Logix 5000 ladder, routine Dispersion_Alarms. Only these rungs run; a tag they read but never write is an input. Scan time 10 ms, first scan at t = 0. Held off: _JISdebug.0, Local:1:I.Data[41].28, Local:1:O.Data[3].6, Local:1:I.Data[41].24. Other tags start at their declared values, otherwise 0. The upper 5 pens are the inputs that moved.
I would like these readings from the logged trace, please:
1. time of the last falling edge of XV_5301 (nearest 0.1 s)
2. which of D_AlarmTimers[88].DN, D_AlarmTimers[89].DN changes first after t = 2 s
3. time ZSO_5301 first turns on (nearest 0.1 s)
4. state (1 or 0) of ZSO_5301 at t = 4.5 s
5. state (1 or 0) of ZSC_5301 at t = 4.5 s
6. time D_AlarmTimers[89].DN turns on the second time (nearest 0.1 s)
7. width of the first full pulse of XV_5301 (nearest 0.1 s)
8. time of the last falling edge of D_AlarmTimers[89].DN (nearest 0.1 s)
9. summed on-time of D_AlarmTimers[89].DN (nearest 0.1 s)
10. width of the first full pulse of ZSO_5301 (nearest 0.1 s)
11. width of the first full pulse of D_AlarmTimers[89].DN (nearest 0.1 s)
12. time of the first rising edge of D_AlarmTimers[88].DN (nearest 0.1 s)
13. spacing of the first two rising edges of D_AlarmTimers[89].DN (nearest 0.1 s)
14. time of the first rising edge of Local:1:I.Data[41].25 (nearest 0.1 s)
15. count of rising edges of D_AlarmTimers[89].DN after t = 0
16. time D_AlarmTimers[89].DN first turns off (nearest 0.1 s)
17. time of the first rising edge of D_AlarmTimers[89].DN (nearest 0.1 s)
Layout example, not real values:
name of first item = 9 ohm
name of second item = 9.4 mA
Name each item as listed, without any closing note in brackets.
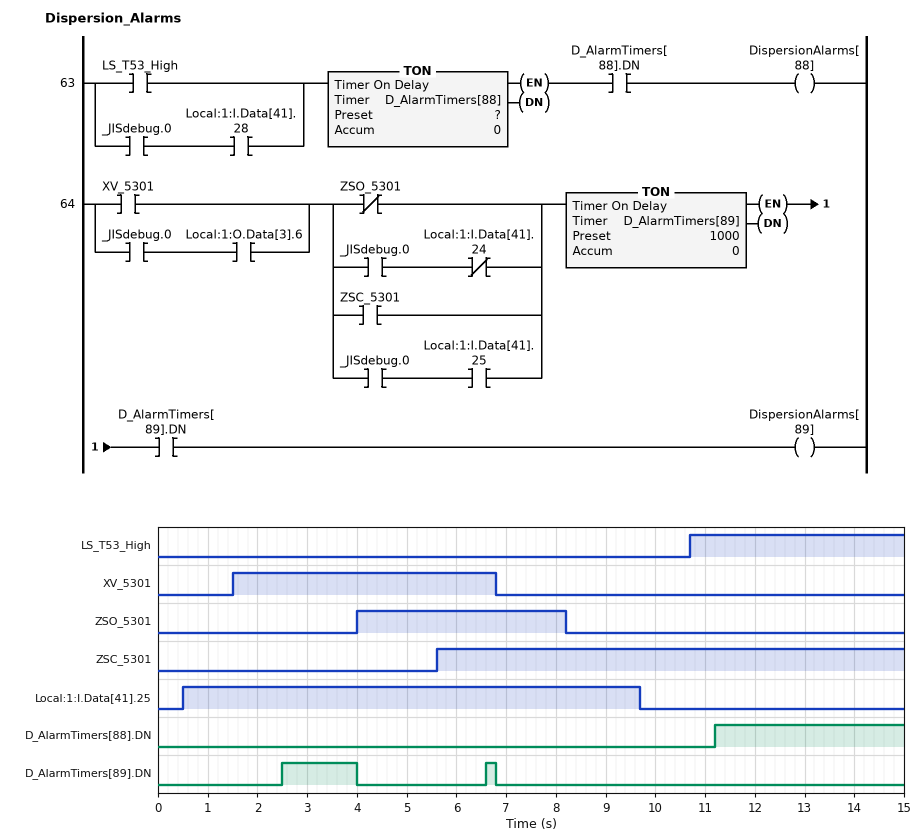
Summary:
time of the last falling edge of XV_5301 = 6.8 s
which of D_AlarmTimers[88].DN, D_AlarmTimers[89].DN changes first after t = 2 s = D_AlarmTimers[89].DN
time ZSO_5301 first turns on = 4.0 s
state (1 or 0) of ZSO_5301 at t = 4.5 s = 1
state (1 or 0) of ZSC_5301 at t = 4.5 s = 0
time D_AlarmTimers[89].DN turns on the second time = 6.6 s
width of the first full pulse of XV_5301 = 5.3 s
time of the last falling edge of D_AlarmTimers[89].DN = 6.8 s
summed on-time of D_AlarmTimers[89].DN = 1.7 s
width of the first full pulse of ZSO_5301 = 4.2 s
width of the first full pulse of D_AlarmTimers[89].DN = 1.5 s
time of the first rising edge of D_AlarmTimers[88].DN = 11.2 s
spacing of the first two rising edges of D_AlarmTimers[89].DN = 4.1 s
time of the first rising edge of Local:1:I.Data[41].25 = 0.5 s
count of rising edges of D_AlarmTimers[89].DN after t = 0 = 2
time D_AlarmTimers[89].DN first turns off = 4.0 s
time of the first rising edge of D_AlarmTimers[89].DN = 2.5 s
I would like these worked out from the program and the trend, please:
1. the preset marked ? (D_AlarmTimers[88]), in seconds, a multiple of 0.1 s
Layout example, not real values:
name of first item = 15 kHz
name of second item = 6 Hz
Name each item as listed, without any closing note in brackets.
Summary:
the preset marked ? (D_AlarmTimers[88]), in seconds, a multiple of 0.1 s = 0.5 s
